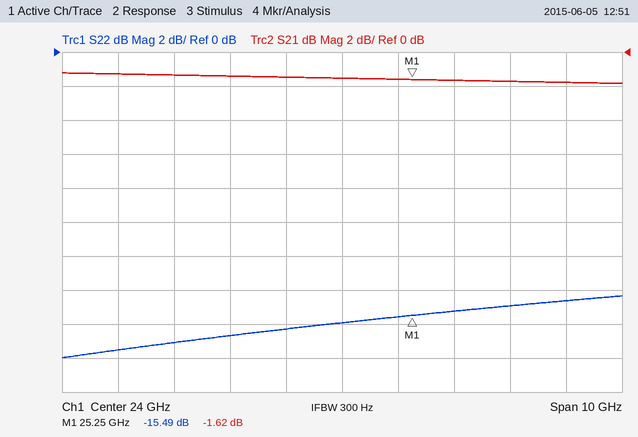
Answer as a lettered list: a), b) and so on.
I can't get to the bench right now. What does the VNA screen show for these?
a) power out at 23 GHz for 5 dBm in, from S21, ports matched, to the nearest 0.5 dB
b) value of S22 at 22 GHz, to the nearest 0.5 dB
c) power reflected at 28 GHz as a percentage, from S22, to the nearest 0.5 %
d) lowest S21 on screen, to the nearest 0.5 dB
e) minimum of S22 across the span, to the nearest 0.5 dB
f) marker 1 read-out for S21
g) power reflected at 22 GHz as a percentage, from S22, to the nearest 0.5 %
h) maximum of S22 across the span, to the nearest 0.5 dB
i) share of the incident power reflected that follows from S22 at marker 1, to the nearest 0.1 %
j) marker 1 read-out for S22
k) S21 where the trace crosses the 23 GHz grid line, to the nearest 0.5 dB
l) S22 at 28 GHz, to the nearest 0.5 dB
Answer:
a) 3.5 dBm
b) -16.5 dB
c) 3.5 %
d) -2.0 dB
e) -18.0 dB
f) -1.62 dB
g) 2.0 %
h) -14.5 dB
i) 2.8 %
j) -15.49 dB
k) -1.5 dB
l) -14.5 dB
